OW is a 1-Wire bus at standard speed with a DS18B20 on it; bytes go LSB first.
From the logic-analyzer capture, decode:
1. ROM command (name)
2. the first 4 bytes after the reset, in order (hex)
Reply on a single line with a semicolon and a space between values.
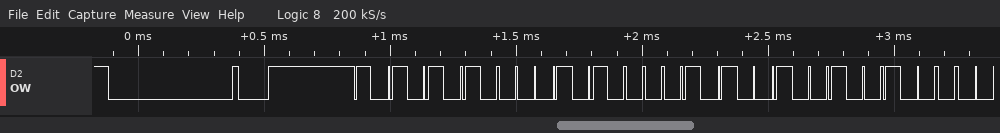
Match ROM; 55 28 94 24
